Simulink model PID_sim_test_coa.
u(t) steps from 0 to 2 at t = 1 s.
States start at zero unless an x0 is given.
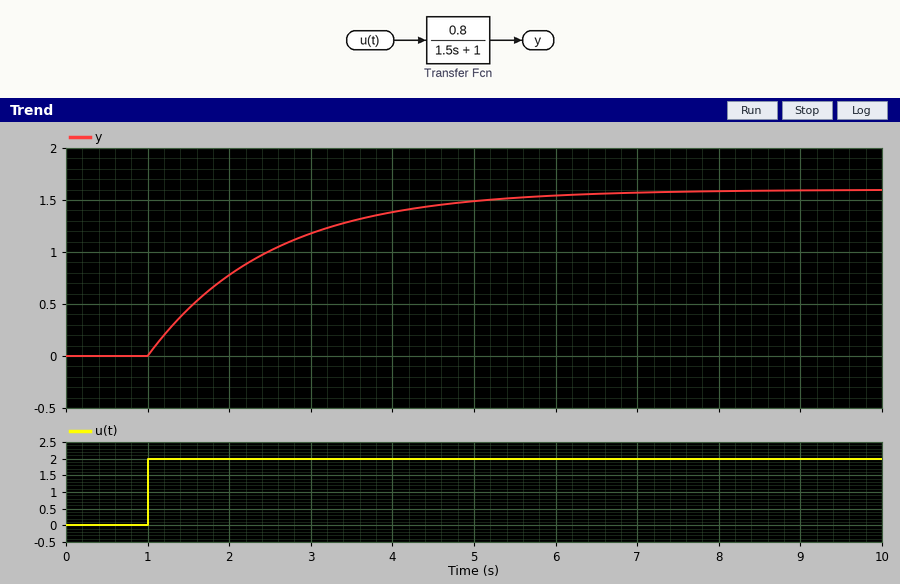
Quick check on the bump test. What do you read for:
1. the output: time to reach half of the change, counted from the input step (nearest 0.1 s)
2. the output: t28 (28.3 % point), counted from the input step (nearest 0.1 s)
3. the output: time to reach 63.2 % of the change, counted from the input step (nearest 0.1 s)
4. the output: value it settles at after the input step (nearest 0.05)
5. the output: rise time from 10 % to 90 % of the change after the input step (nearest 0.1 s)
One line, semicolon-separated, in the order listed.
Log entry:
1.0 s; 0.5 s; 1.5 s; 1.60; 3.3 s
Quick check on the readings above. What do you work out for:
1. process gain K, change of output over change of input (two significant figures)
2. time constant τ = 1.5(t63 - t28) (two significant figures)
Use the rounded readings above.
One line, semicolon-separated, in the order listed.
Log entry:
0.80; 1.5 s
